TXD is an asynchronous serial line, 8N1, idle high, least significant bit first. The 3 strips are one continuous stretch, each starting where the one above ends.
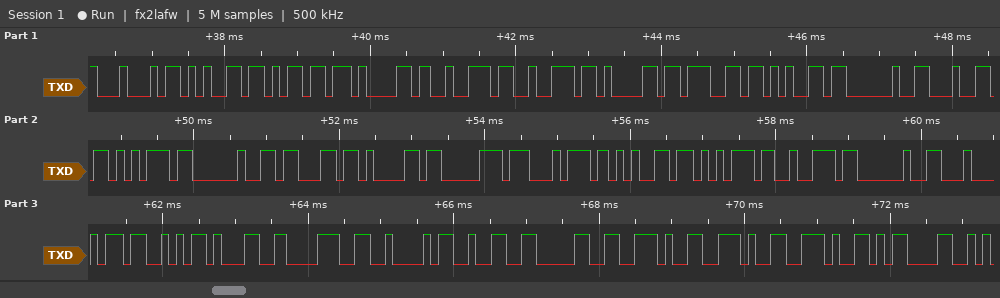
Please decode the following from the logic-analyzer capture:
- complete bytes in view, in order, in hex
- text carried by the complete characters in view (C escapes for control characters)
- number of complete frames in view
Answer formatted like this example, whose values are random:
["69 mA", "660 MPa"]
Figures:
["44 65 6D 61 72 72 61 67 65 20 64 75 20 63 61 70 74 65 75 72 20 44 53 31 38 42 32 30 2E 2E 2E 0D", "\"Demarrage du capteur DS18B20...\\r\"", "32"]
